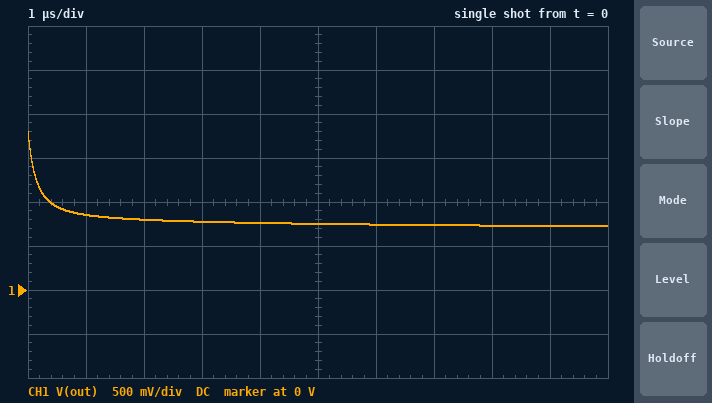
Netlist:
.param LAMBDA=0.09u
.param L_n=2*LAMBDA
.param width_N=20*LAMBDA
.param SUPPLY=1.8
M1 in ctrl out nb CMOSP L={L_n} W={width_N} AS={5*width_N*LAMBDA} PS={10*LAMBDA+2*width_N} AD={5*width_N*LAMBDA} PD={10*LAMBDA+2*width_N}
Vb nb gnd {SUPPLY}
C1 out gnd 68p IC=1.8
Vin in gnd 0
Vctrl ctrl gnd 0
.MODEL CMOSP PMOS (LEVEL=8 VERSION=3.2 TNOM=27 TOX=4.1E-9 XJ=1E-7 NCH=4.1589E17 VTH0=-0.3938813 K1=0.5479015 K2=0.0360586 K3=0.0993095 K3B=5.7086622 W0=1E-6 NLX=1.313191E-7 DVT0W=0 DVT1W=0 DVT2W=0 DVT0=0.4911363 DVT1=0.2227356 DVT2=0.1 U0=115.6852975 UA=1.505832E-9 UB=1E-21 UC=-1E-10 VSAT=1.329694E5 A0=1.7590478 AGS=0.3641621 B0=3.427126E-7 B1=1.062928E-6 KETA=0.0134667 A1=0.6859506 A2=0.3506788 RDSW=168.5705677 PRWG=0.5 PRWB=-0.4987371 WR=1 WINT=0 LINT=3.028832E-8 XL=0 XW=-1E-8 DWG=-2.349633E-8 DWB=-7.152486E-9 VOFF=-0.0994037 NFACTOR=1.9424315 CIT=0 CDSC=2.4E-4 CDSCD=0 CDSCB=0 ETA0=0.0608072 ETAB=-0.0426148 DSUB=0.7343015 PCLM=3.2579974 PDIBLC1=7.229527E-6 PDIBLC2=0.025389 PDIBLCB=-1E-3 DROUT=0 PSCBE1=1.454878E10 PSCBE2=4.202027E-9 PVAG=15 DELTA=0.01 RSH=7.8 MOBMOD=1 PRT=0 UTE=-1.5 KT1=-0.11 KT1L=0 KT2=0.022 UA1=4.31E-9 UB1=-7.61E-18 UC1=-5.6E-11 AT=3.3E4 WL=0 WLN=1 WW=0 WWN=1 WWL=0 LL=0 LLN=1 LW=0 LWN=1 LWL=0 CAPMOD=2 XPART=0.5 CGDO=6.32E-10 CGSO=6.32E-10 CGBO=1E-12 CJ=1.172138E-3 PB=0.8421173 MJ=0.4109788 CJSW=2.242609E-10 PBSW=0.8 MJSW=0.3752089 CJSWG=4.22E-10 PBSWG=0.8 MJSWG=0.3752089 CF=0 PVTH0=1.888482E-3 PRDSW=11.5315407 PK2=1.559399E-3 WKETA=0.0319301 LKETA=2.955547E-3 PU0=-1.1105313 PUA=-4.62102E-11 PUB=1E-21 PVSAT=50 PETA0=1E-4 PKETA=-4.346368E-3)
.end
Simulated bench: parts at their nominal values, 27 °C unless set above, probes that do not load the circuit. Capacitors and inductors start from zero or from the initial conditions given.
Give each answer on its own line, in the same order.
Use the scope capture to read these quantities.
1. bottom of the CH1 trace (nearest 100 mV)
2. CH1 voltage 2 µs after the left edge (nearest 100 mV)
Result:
700 mV
800 mV
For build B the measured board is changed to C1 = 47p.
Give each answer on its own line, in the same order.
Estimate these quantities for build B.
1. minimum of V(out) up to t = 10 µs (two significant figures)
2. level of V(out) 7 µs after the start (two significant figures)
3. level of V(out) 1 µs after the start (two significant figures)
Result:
710 mV
720 mV
820 mV
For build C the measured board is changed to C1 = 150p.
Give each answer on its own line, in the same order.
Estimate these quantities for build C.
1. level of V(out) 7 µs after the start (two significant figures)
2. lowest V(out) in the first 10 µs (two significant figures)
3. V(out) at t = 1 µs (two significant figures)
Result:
770 mV
760 mV
960 mV
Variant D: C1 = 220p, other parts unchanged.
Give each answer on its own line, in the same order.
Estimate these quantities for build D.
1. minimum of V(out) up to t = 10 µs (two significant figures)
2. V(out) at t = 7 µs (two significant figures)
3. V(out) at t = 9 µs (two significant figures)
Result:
770 mV
790 mV
780 mV
